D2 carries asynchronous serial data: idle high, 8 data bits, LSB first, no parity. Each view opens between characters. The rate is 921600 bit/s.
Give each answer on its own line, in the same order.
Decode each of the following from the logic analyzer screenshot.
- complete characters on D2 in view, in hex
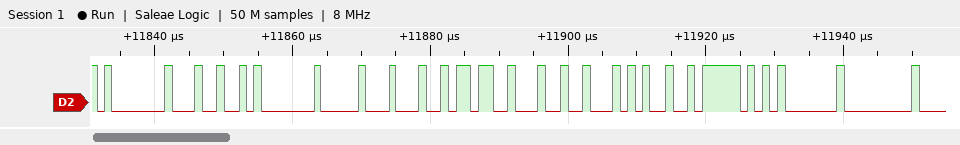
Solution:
01, 24, 01, 10, A4, 13, 12, 25, 5F, 01, 00
